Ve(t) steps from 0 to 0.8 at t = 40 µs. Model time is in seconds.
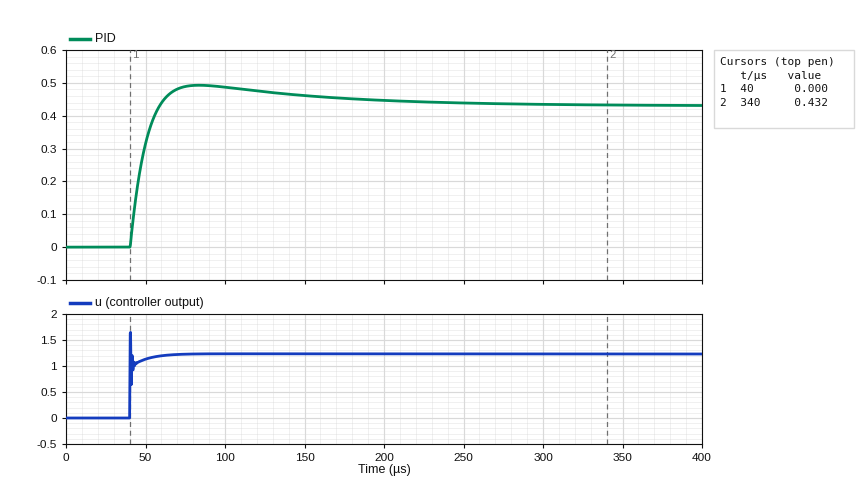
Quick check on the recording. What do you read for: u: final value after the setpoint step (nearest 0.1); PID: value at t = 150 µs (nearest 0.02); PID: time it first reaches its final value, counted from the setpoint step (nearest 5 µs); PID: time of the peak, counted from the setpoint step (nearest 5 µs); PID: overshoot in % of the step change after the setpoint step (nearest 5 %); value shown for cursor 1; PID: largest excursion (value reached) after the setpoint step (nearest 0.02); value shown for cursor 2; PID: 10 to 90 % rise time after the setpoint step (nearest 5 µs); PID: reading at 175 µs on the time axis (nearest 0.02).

1.2
0.46
20 µs
45 µs
15 %
0.000
0.50
0.432
15 µs
0.46
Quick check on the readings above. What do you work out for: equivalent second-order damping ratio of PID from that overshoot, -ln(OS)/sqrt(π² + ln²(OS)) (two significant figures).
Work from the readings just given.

0.52
